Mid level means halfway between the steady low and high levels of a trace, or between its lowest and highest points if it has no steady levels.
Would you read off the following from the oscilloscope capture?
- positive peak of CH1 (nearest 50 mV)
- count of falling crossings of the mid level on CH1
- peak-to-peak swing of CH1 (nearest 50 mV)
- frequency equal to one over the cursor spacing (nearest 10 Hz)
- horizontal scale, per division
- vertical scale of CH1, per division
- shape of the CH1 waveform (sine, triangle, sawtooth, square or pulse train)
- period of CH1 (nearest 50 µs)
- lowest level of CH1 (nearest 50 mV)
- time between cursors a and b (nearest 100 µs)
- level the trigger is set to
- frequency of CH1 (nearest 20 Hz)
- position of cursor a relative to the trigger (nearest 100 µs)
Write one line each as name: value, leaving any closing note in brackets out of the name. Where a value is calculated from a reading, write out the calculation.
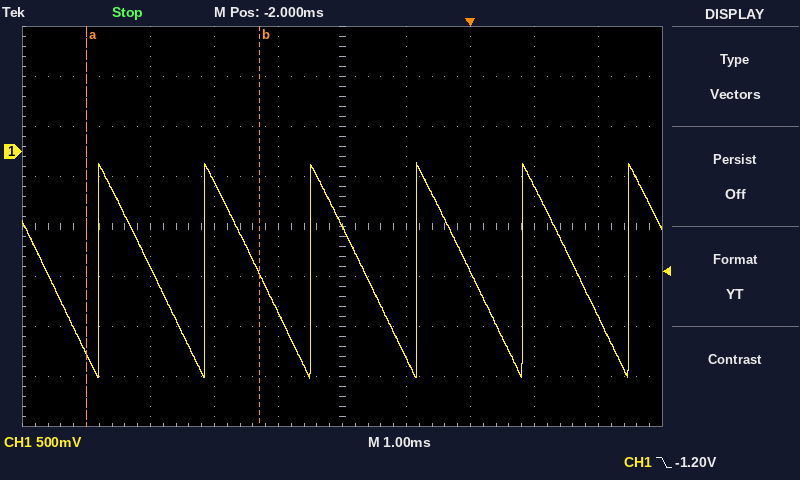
positive peak of CH1: -100 mV
count of falling crossings of the mid level on CH1: 6
peak-to-peak swing of CH1: -100 mV − (-2.25 V) = 2.15 V
frequency equal to one over the cursor spacing: 1 / 2.7 ms ≈ 370 Hz
horizontal scale, per division: 1 ms
vertical scale of CH1, per division: 500 mV
shape of the CH1 waveform: sawtooth
period of CH1: 1.65 ms
lowest level of CH1: -2.25 V
time between cursors a and b: 2.7 ms
level the trigger is set to: -1.20 V
frequency of CH1: 1 / 1.65 ms ≈ 606 Hz, so 600 Hz to the nearest 20 Hz
position of cursor a relative to the trigger: -6.0 ms
